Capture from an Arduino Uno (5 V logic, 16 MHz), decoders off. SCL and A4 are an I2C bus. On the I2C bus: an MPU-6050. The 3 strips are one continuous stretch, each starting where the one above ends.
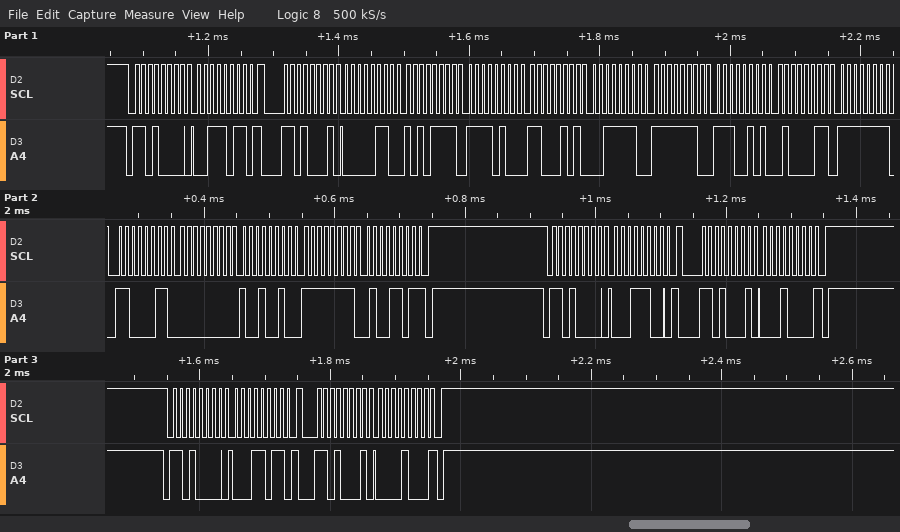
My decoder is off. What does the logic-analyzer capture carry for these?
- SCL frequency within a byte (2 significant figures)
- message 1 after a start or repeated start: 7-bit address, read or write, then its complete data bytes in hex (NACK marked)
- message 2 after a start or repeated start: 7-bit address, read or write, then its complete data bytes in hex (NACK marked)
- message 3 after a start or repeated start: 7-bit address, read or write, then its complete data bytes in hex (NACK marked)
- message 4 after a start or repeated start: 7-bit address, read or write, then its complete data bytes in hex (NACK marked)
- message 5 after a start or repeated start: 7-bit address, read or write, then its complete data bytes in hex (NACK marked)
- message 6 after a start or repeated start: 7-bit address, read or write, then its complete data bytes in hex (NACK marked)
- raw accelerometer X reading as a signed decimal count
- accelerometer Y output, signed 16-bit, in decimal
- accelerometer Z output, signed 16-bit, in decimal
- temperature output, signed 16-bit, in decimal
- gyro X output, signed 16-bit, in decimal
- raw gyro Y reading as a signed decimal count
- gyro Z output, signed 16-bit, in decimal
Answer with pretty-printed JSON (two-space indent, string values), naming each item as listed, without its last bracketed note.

{
  "SCL frequency within a byte": "100 kHz",
  "message 1 after a start or repeated start: 7-bit address, read or write, then its complete data bytes in hex": "0x68 write: 3B",
  "message 2 after a start or repeated start: 7-bit address, read or write, then its complete data bytes in hex": "0x68 read: 06 AF F4 C5 3E FE E5 43 FF C3 00 92 FF 4D NACK",
  "message 3 after a start or repeated start: 7-bit address, read or write, then its complete data bytes in hex": "0x68 write: 1C",
  "message 4 after a start or repeated start: 7-bit address, read or write, then its complete data bytes in hex": "0x68 read: 10 NACK",
  "message 5 after a start or repeated start: 7-bit address, read or write, then its complete data bytes in hex": "0x68 write: 1B",
  "message 6 after a start or repeated start: 7-bit address, read or write, then its complete data bytes in hex": "0x68 read: 08 NACK",
  "raw accelerometer X reading as a signed decimal count": "1711",
  "accelerometer Y output, signed 16-bit, in decimal": "-2875",
  "accelerometer Z output, signed 16-bit, in decimal": "16126",
  "temperature output, signed 16-bit, in decimal": "-6845",
  "gyro X output, signed 16-bit, in decimal": "-61",
  "raw gyro Y reading as a signed decimal count": "146",
  "gyro Z output, signed 16-bit, in decimal": "-179"
}
